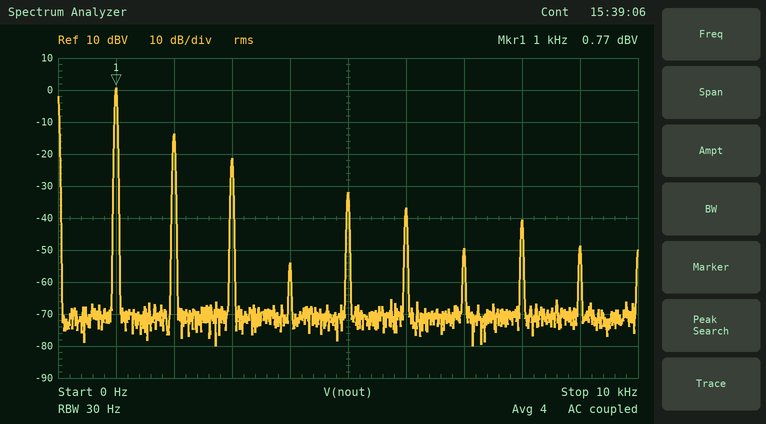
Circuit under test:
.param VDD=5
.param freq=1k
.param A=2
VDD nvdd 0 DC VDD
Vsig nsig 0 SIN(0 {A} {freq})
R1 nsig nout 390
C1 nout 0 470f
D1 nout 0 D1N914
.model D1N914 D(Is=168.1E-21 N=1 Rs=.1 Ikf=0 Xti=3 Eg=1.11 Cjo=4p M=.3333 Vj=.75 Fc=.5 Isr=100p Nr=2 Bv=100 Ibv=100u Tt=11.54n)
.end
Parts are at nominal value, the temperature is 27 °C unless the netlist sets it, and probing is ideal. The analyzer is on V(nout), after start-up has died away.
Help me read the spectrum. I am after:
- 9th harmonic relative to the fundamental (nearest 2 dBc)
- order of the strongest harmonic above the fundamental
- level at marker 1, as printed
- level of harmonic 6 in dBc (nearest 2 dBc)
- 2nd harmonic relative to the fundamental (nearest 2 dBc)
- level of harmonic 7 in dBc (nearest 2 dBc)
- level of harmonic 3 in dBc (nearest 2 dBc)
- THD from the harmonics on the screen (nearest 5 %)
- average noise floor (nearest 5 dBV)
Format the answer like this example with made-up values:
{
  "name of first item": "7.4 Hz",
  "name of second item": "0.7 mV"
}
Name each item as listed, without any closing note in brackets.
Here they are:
{
  "9th harmonic relative to the fundamental": "-50 dBc",
  "order of the strongest harmonic above the fundamental": "2",
  "level at marker 1, as printed": "0.77 dBV",
  "level of harmonic 6 in dBc": "-38 dBc",
  "2nd harmonic relative to the fundamental": "-14 dBc",
  "level of harmonic 7 in dBc": "-50 dBc",
  "level of harmonic 3 in dBc": "-22 dBc",
  "THD from the harmonics on the screen": "20 %",
  "average noise floor": "-70 dBV"
}
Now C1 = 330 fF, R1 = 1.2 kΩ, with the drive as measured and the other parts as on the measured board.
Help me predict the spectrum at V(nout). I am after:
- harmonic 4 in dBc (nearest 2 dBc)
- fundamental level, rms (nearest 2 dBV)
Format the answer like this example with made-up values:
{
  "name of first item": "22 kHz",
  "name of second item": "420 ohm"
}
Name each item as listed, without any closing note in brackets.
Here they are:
{
  "harmonic 4 in dBc": "-52 dBc",
  "fundamental level, rms": "0 dBV"
}
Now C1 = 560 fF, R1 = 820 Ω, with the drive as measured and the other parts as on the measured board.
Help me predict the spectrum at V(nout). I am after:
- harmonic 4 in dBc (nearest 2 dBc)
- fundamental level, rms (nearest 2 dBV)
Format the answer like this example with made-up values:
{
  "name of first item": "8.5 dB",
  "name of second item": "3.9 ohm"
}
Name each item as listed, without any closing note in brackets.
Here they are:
{
  "harmonic 4 in dBc": "-60 dBc",
  "fundamental level, rms": "0 dBV"
}
